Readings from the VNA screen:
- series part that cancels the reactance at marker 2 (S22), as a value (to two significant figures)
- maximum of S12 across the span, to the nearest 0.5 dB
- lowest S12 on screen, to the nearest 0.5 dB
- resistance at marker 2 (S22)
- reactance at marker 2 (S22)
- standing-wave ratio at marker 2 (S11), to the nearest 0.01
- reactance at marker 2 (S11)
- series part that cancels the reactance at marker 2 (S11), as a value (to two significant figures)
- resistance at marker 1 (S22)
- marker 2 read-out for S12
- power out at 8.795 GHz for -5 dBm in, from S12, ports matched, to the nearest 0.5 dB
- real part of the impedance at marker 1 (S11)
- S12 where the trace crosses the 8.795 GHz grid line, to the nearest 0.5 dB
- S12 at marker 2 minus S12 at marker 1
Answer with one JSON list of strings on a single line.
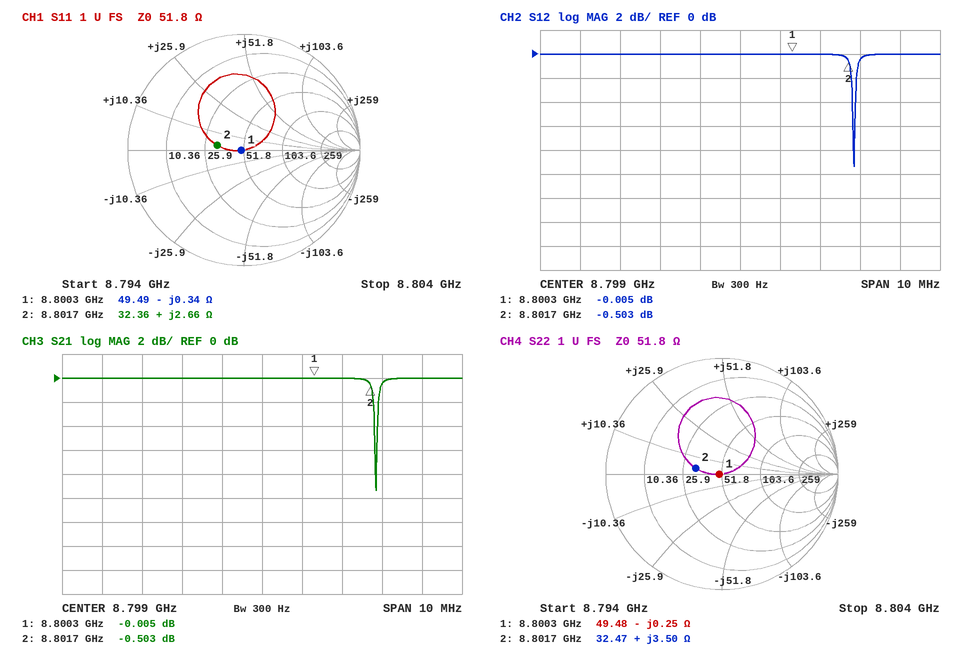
["5.2 pF", "0.0 dB", "-9.5 dB", "32.47 Ω", "+3.50 Ω", "1.61", "+2.66 Ω", "6.8 pF", "49.48 Ω", "-0.503 dB", "-5.0 dBm", "49.49 Ω", "0.0 dB", "-0.498 dB"]
